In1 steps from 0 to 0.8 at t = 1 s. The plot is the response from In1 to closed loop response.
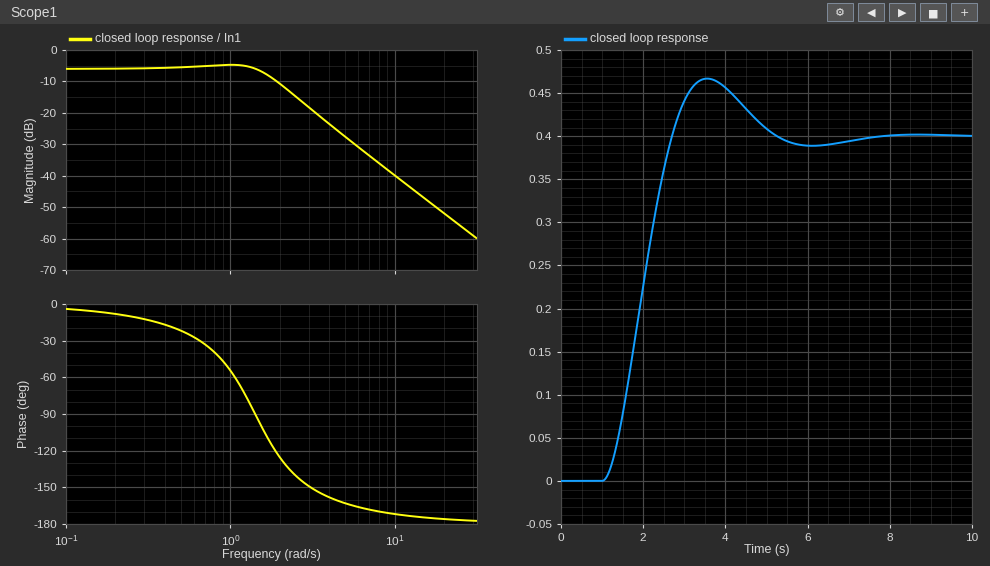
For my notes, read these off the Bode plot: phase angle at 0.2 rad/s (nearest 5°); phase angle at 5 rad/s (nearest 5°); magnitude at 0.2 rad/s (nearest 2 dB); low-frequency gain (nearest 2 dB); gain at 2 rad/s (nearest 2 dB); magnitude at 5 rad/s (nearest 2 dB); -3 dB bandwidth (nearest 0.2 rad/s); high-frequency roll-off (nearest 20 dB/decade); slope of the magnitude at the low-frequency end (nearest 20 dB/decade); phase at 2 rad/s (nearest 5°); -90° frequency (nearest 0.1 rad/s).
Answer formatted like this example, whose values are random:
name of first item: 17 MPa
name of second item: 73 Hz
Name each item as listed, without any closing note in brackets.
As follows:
phase angle at 0.2 rad/s: -10°
phase angle at 5 rad/s: -165°
magnitude at 0.2 rad/s: -6 dB
low-frequency gain: -6 dB
gain at 2 rad/s: -10 dB
magnitude at 5 rad/s: -28 dB
-3 dB bandwidth: 1.8 rad/s
high-frequency roll-off: -40 dB/decade
slope of the magnitude at the low-frequency end: 0 dB/decade
phase at 2 rad/s: -125°
-90° frequency: 1.4 rad/s
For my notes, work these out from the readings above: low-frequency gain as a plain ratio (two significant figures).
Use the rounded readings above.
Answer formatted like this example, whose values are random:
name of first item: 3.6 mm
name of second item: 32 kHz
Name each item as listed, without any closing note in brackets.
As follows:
low-frequency gain as a plain ratio: 0.50
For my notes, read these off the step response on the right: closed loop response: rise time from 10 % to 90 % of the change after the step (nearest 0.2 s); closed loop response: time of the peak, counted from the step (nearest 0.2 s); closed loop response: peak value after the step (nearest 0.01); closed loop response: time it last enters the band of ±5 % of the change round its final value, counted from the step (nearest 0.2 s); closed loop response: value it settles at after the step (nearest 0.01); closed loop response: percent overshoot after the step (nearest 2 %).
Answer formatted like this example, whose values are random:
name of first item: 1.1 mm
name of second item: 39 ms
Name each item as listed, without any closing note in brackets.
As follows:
closed loop response: rise time from 10 % to 90 % of the change after the step: 1.2 s
closed loop response: time of the peak, counted from the step: 2.6 s
closed loop response: peak value after the step: 0.47
closed loop response: time it last enters the band of ±5 % of the change round its final value, counted from the step: 3.8 s
closed loop response: value it settles at after the step: 0.40
closed loop response: percent overshoot after the step: 16 %
